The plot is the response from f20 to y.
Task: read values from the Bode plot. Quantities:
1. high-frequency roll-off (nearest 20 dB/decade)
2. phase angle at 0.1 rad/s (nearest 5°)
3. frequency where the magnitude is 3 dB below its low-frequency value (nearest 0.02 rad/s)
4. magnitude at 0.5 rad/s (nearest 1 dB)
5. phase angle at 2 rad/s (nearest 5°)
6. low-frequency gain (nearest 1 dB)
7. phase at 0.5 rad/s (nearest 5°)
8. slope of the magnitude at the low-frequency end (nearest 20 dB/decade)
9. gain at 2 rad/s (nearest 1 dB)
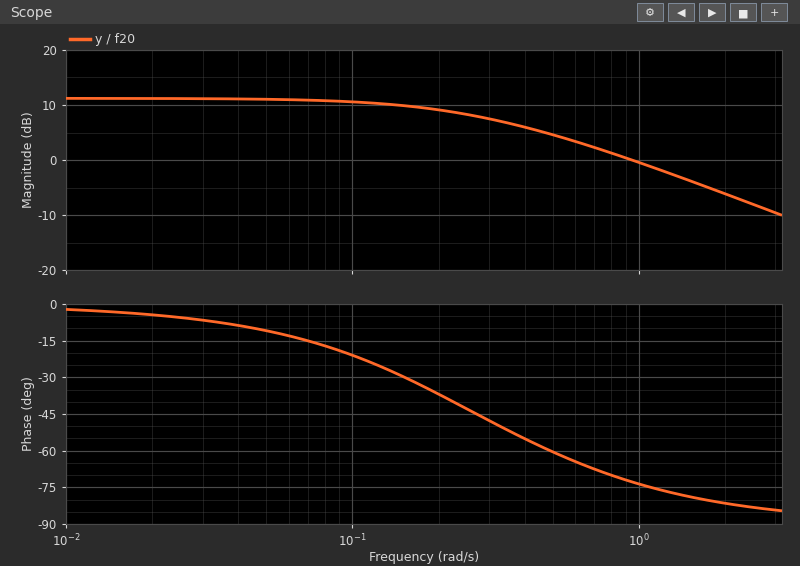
-20 dB/decade
-20°
0.26 rad/s
5 dB
-80°
11 dB
-60°
0 dB/decade
-6 dB
